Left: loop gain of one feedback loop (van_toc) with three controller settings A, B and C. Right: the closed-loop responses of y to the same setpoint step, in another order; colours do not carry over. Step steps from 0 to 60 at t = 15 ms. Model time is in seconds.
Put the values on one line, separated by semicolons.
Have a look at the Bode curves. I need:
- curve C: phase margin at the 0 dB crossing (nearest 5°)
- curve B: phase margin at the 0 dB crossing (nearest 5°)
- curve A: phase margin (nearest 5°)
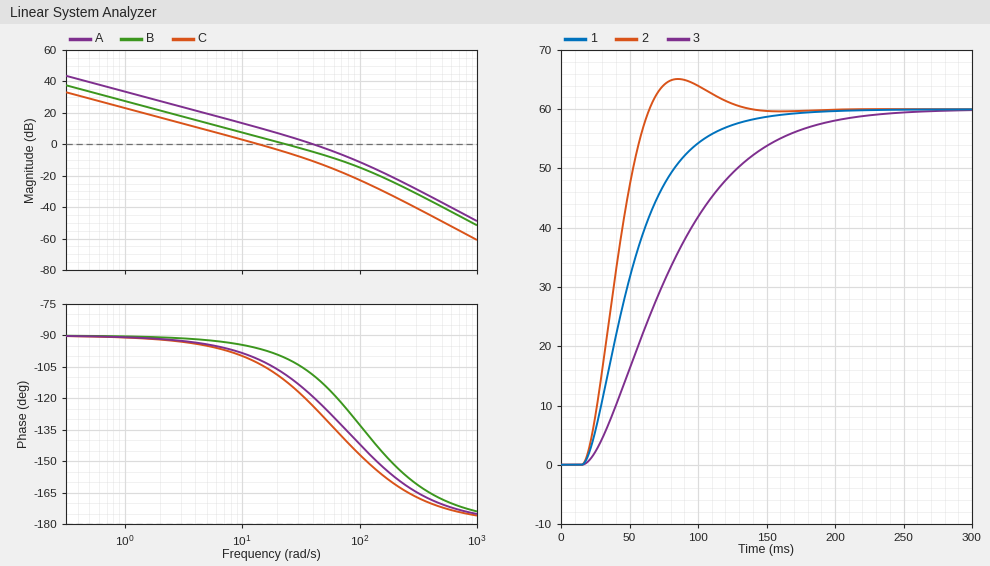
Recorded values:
75°; 80°; 60°
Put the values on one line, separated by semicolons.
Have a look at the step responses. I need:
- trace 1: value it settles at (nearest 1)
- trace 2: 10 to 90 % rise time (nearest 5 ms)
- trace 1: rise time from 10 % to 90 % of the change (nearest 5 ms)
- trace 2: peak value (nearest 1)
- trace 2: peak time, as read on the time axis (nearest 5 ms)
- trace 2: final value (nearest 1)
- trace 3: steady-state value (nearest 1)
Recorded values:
60; 35 ms; 75 ms; 65; 85 ms; 60; 60
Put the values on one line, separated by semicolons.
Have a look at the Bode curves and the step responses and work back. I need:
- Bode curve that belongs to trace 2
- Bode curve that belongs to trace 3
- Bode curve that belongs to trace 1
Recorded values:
A; C; B
